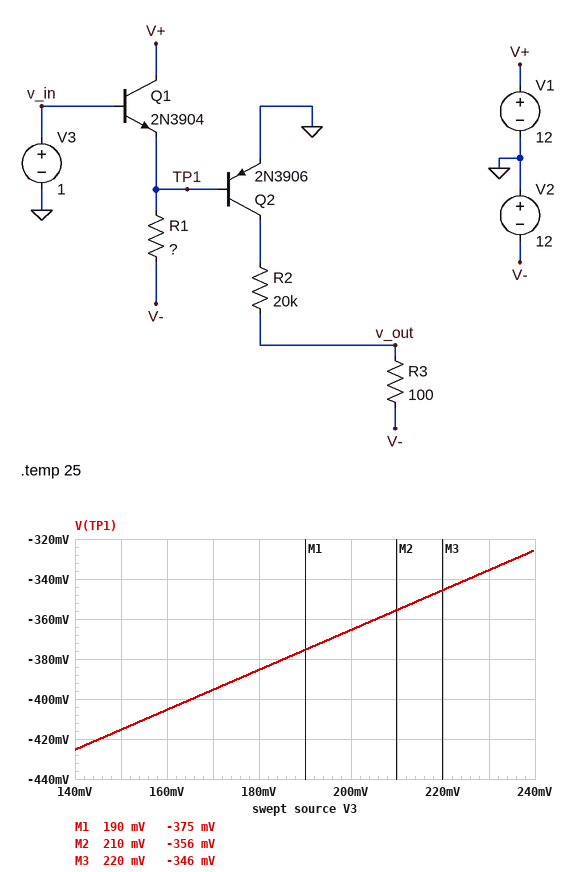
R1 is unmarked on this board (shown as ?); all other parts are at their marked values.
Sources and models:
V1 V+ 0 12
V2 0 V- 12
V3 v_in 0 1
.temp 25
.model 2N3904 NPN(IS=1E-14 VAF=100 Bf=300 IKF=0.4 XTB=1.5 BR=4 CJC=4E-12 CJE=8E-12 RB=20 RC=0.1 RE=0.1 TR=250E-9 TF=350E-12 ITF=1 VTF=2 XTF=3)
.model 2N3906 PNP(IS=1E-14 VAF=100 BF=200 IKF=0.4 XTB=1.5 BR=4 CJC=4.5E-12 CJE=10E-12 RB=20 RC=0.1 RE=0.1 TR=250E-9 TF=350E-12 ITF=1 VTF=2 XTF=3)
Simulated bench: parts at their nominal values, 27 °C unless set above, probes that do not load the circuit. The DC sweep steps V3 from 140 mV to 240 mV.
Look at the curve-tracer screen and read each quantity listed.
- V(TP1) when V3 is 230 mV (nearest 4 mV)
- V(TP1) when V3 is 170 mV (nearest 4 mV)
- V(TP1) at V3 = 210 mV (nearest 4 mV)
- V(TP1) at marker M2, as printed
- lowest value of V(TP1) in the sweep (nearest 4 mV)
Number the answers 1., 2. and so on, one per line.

1. -336 mV
2. -396 mV
3. -356 mV
4. -356 mV
5. -424 mV
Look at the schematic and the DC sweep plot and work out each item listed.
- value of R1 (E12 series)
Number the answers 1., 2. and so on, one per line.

1. 390 kΩ
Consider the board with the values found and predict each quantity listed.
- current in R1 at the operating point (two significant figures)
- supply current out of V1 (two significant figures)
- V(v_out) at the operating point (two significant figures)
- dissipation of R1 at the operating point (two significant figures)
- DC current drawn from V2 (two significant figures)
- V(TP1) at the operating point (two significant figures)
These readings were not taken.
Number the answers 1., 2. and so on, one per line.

1. 32 µA
2. 32 µA
3. -12 V
4. 400 µW
5. 32 µA
6. 430 mV
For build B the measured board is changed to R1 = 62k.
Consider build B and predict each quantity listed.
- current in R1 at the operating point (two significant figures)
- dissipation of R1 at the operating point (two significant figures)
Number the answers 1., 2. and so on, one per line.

1. 200 µA
2. 2.5 mW
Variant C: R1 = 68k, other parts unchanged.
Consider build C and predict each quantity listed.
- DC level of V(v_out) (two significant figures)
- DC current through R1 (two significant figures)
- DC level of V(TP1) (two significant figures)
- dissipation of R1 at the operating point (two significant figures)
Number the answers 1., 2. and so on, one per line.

1. -12 V
2. 180 µA
3. 390 mV
4. 2.3 mW
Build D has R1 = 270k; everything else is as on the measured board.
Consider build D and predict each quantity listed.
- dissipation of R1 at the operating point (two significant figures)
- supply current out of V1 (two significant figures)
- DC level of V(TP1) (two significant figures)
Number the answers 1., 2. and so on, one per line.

1. 570 µW
2. 46 µA
3. 420 mV
